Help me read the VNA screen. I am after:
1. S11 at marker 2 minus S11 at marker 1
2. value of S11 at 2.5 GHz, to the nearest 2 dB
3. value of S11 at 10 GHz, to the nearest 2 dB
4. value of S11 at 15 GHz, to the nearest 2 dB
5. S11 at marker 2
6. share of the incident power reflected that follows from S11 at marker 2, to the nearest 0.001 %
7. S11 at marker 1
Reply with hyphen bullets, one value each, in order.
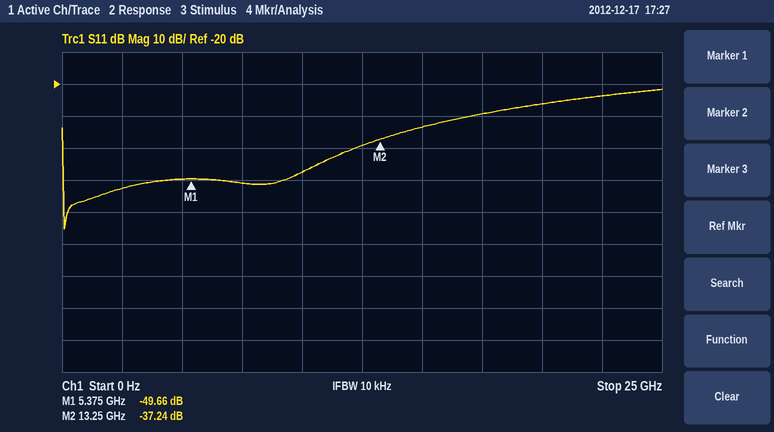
- 12.42 dB
- -52 dB
- -48 dB
- -34 dB
- -37.24 dB
- 0.019 %
- -49.66 dB
